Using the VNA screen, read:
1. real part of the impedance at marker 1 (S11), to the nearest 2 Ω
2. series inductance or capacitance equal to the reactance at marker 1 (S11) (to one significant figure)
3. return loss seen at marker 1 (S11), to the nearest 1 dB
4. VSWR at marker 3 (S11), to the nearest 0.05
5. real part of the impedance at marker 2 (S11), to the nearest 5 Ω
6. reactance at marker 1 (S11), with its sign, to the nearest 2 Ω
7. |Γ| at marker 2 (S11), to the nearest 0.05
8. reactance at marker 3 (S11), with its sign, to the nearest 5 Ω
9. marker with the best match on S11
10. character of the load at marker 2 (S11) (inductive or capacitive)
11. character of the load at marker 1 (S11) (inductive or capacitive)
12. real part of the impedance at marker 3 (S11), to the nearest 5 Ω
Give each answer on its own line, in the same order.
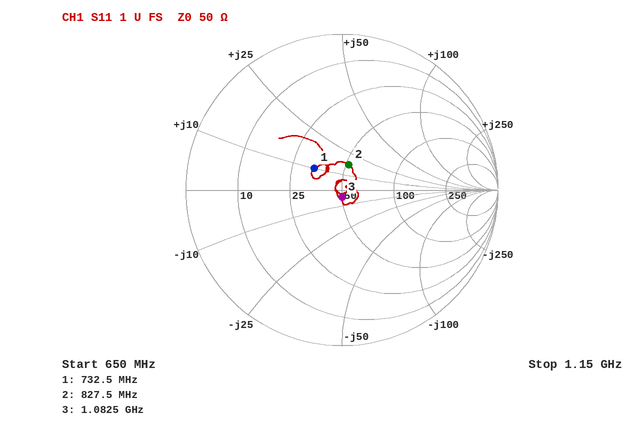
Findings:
34 Ω
2 nH
13 dB
1.10
50 Ω
+10 Ω
0.15
-5 Ω
marker 3
inductive
inductive
50 Ω
